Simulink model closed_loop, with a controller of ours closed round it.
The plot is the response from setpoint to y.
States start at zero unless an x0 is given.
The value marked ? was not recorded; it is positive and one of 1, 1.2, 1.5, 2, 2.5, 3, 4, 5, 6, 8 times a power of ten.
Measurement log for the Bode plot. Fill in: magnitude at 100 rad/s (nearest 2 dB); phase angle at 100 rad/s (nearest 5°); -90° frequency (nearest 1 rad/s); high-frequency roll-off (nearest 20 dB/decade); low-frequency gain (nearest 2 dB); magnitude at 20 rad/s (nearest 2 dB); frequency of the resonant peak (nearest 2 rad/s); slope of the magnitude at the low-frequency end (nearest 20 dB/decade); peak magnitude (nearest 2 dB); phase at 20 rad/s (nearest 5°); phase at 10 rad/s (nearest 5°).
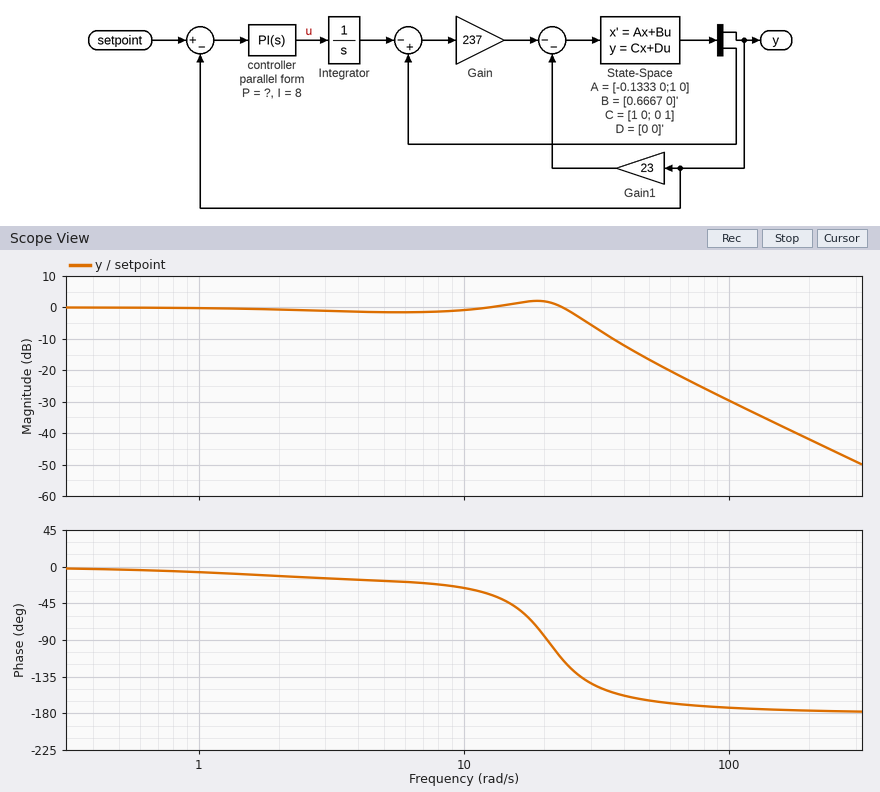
-30 dB
-175°
21 rad/s
-40 dB/decade
0 dB
2 dB
18 rad/s
0 dB/decade
2 dB
-85°
-25°
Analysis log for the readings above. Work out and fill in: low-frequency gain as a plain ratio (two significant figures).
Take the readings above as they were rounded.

1.0
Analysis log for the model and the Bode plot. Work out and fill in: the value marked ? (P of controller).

2
